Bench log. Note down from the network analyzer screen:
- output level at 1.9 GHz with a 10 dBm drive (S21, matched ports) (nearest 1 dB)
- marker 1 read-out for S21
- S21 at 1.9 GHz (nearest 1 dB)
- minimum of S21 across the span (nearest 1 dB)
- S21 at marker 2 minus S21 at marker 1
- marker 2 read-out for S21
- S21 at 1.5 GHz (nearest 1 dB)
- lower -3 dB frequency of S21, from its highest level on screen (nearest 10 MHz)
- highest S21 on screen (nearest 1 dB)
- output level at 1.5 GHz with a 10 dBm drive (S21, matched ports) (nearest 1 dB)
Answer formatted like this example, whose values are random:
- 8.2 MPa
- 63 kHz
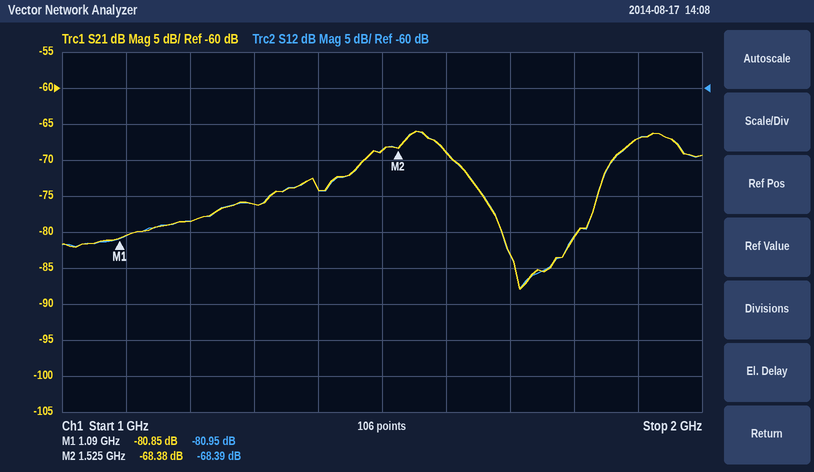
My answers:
- -57 dBm
- -80.85 dB
- -67 dB
- -88 dB
- 12.47 dB
- -68.38 dB
- -69 dB
- 1.48 GHz
- -66 dB
- -59 dBm
